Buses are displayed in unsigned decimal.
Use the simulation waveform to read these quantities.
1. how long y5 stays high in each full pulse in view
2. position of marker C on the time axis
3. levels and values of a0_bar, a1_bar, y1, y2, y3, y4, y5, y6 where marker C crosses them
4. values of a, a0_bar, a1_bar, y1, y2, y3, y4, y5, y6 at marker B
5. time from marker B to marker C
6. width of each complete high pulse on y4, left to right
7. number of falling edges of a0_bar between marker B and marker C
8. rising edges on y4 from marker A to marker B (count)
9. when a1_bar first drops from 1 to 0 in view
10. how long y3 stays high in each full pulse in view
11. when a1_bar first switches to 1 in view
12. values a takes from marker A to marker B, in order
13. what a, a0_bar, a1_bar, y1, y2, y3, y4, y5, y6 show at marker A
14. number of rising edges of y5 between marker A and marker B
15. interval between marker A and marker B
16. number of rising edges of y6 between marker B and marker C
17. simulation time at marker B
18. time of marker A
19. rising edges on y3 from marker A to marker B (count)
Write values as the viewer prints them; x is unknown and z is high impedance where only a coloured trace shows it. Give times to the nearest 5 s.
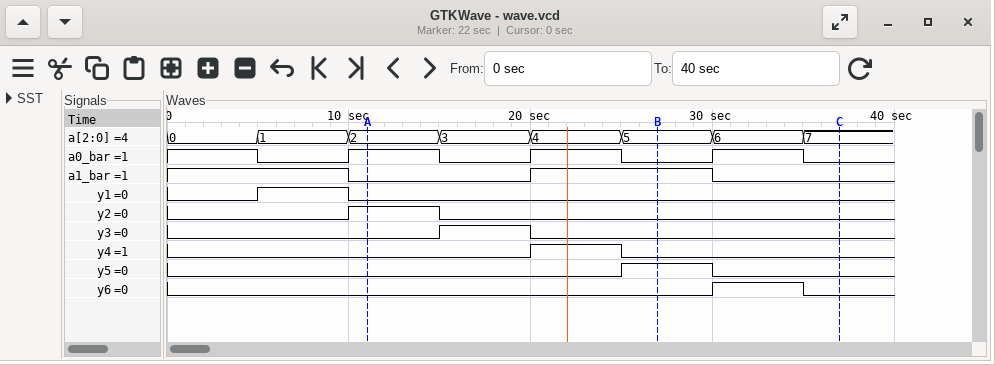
5 s
35 s
a0_bar=0, a1_bar=0, y1=0, y2=0, y3=0, y4=0, y5=0, y6=0
a=5, a0_bar=0, a1_bar=1, y1=0, y2=0, y3=0, y4=0, y5=1, y6=0
10 s
5 s
1
1
10 s
5 s
20 s
2, 3, 4, 5
a=2, a0_bar=1, a1_bar=0, y1=0, y2=1, y3=0, y4=0, y5=0, y6=0
1
15 s
1
25 s
10 s
1
